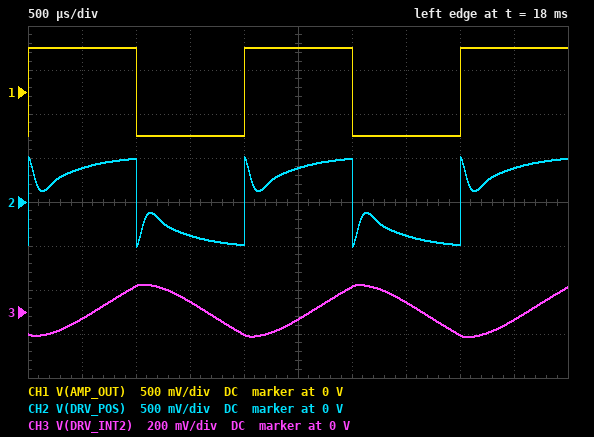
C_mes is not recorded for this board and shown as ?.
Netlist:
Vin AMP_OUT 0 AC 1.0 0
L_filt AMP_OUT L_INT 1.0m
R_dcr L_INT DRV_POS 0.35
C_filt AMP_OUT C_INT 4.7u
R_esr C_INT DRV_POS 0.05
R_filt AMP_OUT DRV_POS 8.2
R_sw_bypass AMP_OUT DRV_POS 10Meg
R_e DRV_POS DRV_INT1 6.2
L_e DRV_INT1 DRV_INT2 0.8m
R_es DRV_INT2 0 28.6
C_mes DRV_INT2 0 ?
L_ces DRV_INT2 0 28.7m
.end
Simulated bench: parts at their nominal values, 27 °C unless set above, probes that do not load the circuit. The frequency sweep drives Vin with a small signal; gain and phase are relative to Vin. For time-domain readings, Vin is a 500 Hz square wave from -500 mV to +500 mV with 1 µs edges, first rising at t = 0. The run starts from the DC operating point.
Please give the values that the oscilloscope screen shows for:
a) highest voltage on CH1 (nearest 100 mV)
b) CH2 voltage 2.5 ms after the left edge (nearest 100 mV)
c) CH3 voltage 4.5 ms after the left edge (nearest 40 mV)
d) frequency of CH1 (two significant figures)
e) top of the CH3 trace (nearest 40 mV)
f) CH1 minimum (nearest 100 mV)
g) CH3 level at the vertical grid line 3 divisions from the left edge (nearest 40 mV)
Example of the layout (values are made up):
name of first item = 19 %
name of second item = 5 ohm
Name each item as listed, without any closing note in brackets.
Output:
highest voltage on CH1 = 500 mV
CH2 voltage 2.5 ms after the left edge = 400 mV
CH3 voltage 4.5 ms after the left edge = -40 mV
frequency of CH1 = 500 Hz
top of the CH3 trace = 120 mV
CH1 minimum = -500 mV
CH3 level at the vertical grid line 3 divisions from the left edge = 40 mV
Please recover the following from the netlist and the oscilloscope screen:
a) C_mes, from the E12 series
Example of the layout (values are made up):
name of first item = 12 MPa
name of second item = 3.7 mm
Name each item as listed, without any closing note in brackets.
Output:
C_mes, from the E12 series = 220 µF
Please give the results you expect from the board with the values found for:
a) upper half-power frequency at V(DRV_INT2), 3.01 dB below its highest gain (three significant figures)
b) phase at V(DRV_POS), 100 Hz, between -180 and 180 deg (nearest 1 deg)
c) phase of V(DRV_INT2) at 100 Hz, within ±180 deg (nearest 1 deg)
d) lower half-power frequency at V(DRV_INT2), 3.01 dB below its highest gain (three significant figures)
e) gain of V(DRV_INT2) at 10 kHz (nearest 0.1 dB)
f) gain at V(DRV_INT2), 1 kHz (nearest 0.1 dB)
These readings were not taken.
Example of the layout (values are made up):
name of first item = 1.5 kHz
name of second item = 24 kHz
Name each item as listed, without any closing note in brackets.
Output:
upper half-power frequency at V(DRV_INT2), 3.01 dB below its highest gain = 181 Hz
phase at V(DRV_POS), 100 Hz, between -180 and 180 deg = -3 deg
phase of V(DRV_INT2) at 100 Hz, within ±180 deg = -27 deg
lower half-power frequency at V(DRV_INT2), 3.01 dB below its highest gain = 25.7 Hz
gain of V(DRV_INT2) at 10 kHz = -56.4 dB
gain at V(DRV_INT2), 1 kHz = -25.0 dB
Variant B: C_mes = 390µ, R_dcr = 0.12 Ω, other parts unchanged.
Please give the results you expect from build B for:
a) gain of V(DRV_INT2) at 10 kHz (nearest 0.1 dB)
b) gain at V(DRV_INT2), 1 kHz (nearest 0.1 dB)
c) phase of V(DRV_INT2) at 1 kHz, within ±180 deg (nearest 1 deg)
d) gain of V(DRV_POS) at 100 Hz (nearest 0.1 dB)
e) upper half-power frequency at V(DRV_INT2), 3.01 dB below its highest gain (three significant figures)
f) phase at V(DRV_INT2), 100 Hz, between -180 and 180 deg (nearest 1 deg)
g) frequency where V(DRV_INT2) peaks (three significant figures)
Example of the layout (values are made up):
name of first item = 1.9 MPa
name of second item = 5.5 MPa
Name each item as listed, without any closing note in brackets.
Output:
gain of V(DRV_INT2) at 10 kHz = -61.4 dB
gain at V(DRV_INT2), 1 kHz = -30.2 dB
phase of V(DRV_INT2) at 1 kHz, within ±180 deg = -130 deg
gain of V(DRV_POS) at 100 Hz = 0.2 dB
upper half-power frequency at V(DRV_INT2), 3.01 dB below its highest gain = 110 Hz
phase at V(DRV_INT2), 100 Hz, between -180 and 180 deg = -51 deg
frequency where V(DRV_INT2) peaks = 50.7 Hz
